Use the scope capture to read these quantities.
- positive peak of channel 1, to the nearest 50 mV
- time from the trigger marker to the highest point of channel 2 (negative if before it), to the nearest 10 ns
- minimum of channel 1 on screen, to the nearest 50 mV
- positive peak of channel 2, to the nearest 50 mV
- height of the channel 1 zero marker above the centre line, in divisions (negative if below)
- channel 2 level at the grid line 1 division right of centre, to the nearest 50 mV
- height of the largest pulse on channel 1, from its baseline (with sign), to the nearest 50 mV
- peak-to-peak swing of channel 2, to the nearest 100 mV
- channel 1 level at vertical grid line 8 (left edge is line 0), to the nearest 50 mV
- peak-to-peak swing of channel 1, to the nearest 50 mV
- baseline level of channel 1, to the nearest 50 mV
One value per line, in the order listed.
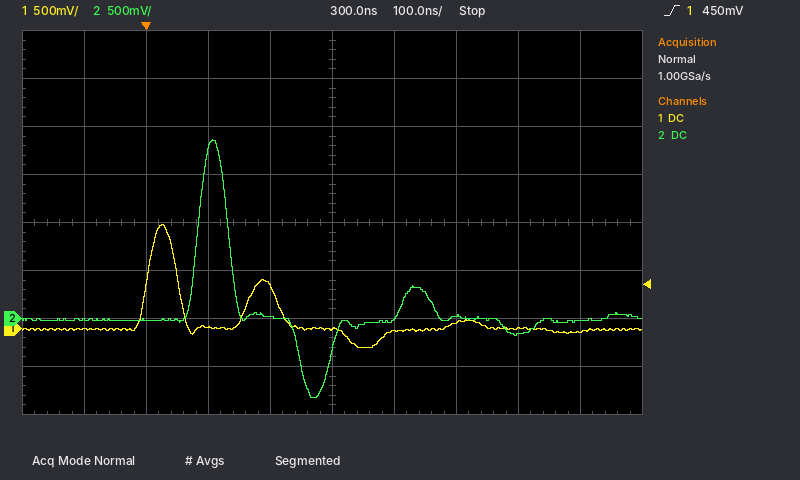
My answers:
1.10 V
+110 ns
-200 mV
1.85 V
-2.2 div
0 mV
+1.10 V
2.70 V
0 mV
1.30 V
0 mV
